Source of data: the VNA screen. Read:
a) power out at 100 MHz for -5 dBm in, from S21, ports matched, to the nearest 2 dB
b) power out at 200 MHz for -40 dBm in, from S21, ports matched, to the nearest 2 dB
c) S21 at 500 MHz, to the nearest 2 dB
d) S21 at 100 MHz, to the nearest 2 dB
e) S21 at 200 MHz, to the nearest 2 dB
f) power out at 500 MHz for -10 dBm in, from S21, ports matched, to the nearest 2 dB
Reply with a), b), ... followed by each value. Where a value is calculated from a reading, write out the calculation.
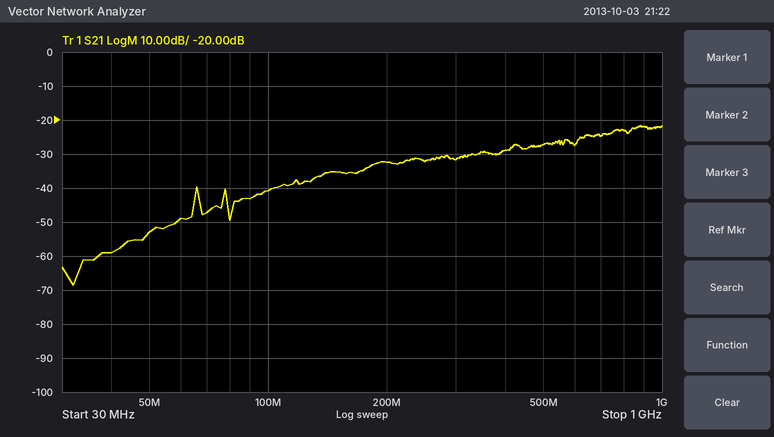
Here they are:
a) -5 dBm + (-40 dB) = -46 dBm
b) -40 dBm + (-32 dB) = -72 dBm
c) -28 dB
d) -40 dB
e) -32 dB
f) -10 dBm + (-28 dB) = -38 dBm
